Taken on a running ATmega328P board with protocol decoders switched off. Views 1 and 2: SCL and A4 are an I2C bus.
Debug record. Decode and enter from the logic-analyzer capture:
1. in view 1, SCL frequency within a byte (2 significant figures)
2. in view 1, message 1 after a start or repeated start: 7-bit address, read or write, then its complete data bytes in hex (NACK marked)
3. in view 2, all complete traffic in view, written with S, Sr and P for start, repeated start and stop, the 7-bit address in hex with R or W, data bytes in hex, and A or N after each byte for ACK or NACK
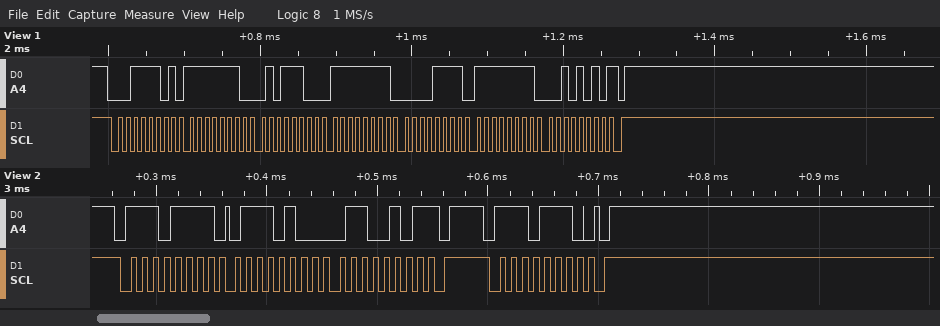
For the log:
100 kHz
0x1E read: FE 5C FF 0F FF 2A NACK
S 77R A 74 A 65 N P S 77W A P
